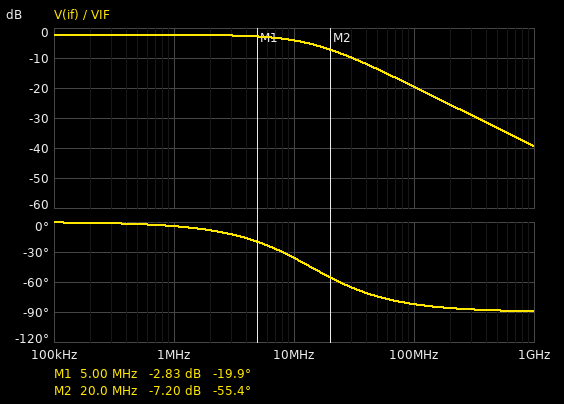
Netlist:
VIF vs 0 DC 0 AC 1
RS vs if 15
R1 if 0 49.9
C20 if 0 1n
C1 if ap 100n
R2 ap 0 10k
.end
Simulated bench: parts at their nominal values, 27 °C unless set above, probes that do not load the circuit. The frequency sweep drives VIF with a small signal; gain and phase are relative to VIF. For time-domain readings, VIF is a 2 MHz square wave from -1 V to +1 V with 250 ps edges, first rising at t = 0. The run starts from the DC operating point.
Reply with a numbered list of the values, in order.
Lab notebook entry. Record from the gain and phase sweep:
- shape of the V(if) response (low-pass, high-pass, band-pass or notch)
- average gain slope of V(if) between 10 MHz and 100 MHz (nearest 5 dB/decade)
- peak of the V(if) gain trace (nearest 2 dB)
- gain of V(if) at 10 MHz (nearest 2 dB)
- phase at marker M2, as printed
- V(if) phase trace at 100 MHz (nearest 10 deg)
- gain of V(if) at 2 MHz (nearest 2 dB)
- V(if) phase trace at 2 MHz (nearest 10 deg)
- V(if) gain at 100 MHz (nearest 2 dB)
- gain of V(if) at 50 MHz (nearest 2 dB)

1. low-pass
2. -15 dB/decade
3. -2 dB
4. -4 dB
5. -55.4 deg
6. -80 deg
7. -2 dB
8. -10 deg
9. -20 dB
10. -14 dB
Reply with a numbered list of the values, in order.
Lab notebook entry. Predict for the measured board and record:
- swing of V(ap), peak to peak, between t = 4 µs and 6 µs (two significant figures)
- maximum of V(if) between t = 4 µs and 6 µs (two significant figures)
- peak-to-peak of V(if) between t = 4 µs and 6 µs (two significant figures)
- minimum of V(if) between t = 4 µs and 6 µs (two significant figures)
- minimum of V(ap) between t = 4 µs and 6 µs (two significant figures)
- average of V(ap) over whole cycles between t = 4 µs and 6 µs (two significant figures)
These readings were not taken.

1. 1.5 V
2. 770 mV
3. 1.5 V
4. -770 mV
5. -4.6 mV
6. 760 mV
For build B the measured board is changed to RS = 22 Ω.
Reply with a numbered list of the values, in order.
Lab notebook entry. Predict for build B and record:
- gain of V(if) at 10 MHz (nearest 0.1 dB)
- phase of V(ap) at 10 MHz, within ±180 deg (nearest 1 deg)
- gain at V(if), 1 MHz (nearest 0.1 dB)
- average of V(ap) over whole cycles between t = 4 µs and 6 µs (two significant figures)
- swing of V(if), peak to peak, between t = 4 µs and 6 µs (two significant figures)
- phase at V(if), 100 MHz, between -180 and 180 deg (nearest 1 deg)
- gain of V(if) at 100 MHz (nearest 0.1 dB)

1. -6.0 dB
2. -44 deg
3. -3.2 dB
4. 690 mV
5. 1.4 V
6. -84 deg
7. -22.9 dB
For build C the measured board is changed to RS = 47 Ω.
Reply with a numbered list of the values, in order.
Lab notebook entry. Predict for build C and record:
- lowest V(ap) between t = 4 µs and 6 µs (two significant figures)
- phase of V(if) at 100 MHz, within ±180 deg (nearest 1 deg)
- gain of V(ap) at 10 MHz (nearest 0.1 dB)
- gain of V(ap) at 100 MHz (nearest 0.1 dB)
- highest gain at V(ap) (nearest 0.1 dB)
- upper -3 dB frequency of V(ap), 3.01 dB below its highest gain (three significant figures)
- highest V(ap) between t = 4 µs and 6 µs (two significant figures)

1. -3.0 mV
2. -86 deg
3. -11.0 dB
4. -29.4 dB
5. -5.8 dB
6. 6.59 MHz
7. 1.0 V
